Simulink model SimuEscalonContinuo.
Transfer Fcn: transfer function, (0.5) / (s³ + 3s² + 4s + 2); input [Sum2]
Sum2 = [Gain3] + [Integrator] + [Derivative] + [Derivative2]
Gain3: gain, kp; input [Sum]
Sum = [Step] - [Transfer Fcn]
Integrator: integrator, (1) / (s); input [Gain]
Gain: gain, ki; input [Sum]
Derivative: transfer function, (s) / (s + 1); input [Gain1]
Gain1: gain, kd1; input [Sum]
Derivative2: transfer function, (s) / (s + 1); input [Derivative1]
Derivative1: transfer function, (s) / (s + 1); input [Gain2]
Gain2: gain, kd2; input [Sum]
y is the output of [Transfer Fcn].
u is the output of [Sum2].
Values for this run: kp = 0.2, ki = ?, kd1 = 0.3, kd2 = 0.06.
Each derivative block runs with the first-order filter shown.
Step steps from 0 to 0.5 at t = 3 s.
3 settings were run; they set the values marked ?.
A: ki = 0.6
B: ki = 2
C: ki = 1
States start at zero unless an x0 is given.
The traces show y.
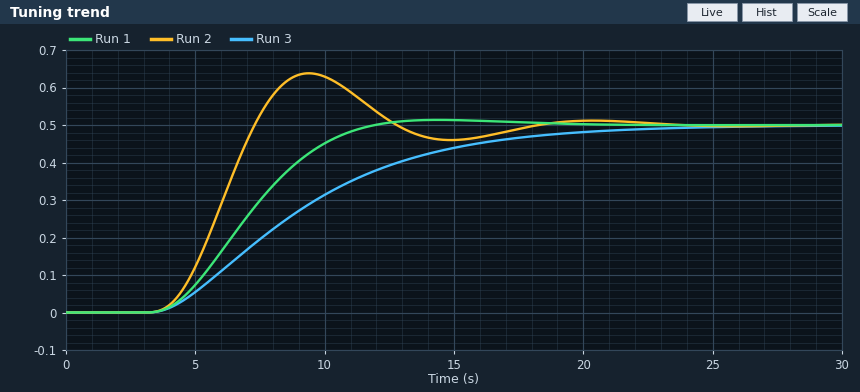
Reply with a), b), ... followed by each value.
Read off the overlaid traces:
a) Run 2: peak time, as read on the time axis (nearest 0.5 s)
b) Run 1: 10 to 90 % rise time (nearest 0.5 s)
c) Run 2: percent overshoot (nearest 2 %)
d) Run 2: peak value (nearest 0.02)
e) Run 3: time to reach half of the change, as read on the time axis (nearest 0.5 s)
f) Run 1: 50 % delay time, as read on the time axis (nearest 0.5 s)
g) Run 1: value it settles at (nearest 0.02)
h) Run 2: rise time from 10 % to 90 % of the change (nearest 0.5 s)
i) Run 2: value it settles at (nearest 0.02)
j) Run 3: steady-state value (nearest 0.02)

a) 9.5 s
b) 5.5 s
c) 28 %
d) 0.64
e) 8.5 s
f) 7.0 s
g) 0.50
h) 2.5 s
i) 0.50
j) 0.50
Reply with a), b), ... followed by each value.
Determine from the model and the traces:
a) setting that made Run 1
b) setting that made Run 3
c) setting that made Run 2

a) C
b) A
c) B
